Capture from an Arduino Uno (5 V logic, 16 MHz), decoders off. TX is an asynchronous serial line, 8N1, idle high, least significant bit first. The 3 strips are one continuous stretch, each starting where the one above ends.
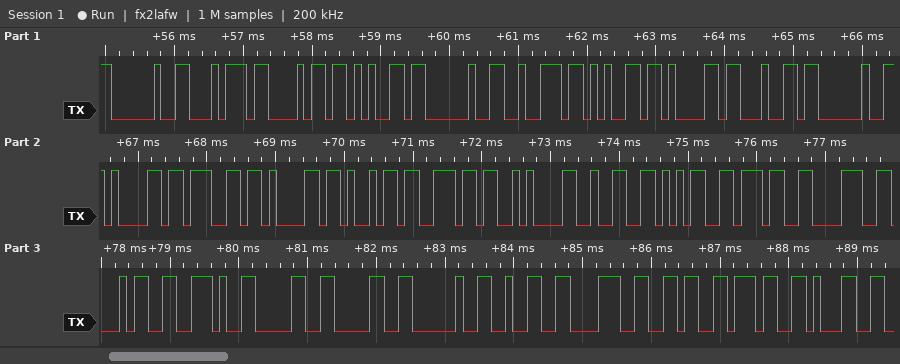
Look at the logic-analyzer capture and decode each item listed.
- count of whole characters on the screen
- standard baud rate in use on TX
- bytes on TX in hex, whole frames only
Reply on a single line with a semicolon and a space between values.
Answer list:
30; 9600 baud; 20 74 68 65 20 72 65 61 64 20 61 67 61 69 6E 0A 32 35 37 38 34 2E 30 30 20 32 38 36 37 31
